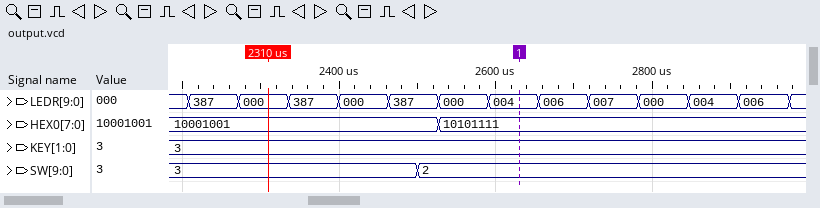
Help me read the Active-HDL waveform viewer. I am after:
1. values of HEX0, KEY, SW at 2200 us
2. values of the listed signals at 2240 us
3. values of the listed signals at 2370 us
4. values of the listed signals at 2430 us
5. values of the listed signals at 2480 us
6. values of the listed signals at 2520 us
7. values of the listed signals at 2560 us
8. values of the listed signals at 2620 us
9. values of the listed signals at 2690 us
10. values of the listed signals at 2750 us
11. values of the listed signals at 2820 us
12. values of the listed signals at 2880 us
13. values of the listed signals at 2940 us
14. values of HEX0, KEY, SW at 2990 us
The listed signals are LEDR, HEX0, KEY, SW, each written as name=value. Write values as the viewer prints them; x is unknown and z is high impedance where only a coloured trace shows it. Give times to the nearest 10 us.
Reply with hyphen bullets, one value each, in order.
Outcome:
- HEX0=10001001, KEY=3, SW=3
- LEDR=387, HEX0=10001001, KEY=3, SW=3
- LEDR=387, HEX0=10001001, KEY=3, SW=3
- LEDR=000, HEX0=10001001, KEY=3, SW=3
- LEDR=387, HEX0=10001001, KEY=3, SW=3
- LEDR=387, HEX0=10001001, KEY=3, SW=2
- LEDR=000, HEX0=10101111, KEY=3, SW=2
- LEDR=004, HEX0=10101111, KEY=3, SW=2
- LEDR=006, HEX0=10101111, KEY=3, SW=2
- LEDR=007, HEX0=10101111, KEY=3, SW=2
- LEDR=000, HEX0=10101111, KEY=3, SW=2
- LEDR=004, HEX0=10101111, KEY=3, SW=2
- LEDR=006, HEX0=10101111, KEY=3, SW=2
- HEX0=10101111, KEY=3, SW=2
